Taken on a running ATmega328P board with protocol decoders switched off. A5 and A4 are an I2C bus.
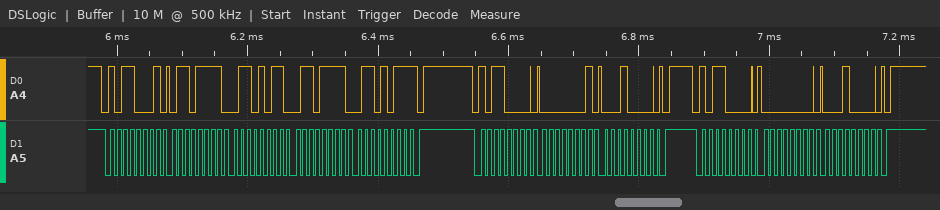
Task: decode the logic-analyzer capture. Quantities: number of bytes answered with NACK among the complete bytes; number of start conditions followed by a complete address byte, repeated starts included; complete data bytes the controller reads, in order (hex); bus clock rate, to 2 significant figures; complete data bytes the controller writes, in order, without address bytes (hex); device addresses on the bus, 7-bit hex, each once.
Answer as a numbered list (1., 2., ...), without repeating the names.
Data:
1. 1
2. 3
3. 6F 6B 6F 6B
4. 100 kHz
5. 01 10 00 10
6. 0x58
